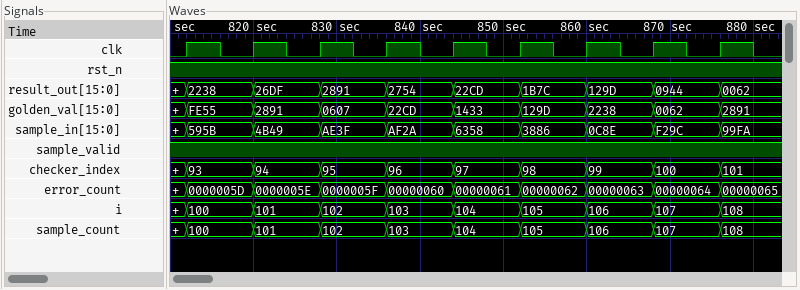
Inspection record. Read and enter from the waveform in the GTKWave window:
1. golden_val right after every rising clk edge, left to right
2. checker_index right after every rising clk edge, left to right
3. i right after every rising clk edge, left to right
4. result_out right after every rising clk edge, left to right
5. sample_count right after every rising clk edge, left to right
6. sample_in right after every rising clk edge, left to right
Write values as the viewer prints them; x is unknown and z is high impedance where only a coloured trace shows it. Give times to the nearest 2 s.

FE55, 2891, 0607, 22CD, 1433, 129D, 2238, 0062, 2891
93, 94, 95, 96, 97, 98, 99, 100, 101
100, 101, 102, 103, 104, 105, 106, 107, 108
2238, 26DF, 2891, 2754, 22CD, 1B7C, 129D, 0944, 0062
100, 101, 102, 103, 104, 105, 106, 107, 108
595B, 4B49, AE3F, AF2A, 6358, 3886, 0C8E, F29C, 99FA
